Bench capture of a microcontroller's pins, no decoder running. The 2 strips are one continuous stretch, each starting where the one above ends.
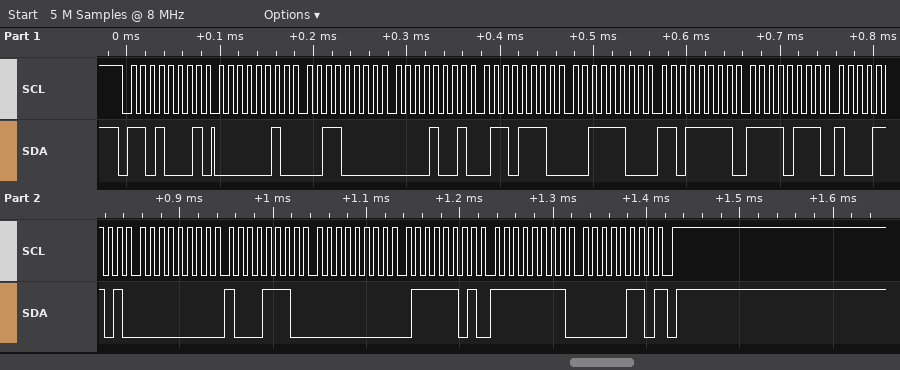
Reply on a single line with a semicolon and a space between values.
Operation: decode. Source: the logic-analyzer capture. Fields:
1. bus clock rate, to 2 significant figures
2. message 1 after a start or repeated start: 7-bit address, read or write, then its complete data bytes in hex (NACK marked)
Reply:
100 kHz; 0x68 read: 02 30 09 6E 3C DF F7 8D 00 8E 00 7D FF 06 NACK
